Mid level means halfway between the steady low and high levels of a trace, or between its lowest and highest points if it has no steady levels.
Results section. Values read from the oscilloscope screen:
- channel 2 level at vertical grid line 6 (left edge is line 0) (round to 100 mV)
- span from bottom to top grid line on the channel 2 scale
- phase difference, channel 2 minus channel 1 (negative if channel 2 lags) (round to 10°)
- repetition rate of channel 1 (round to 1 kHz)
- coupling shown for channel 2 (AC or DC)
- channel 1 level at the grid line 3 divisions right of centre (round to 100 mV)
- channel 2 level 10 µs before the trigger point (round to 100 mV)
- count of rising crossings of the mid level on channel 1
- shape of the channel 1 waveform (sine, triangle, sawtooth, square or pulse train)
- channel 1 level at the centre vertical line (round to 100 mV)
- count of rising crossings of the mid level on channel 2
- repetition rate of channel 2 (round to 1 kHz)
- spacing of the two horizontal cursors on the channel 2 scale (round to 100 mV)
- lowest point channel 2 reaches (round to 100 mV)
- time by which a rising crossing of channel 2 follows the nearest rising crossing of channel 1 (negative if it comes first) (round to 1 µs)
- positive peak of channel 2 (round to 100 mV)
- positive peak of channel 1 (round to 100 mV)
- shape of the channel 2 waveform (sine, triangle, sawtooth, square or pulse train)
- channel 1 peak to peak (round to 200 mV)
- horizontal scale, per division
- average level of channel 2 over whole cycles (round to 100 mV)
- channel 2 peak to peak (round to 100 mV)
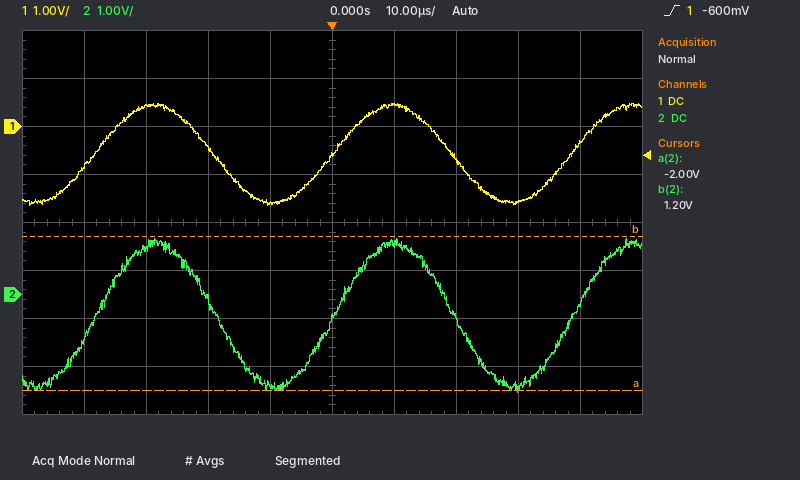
1.1 V
8 V
0°
26 kHz
DC
-1.6 V
-1.9 V
3
sine
-600 mV
3
26 kHz
3.2 V
-2.0 V
0 µs
1.2 V
500 mV
sine
2.2 V
10 µs
-400 mV
3.2 V
